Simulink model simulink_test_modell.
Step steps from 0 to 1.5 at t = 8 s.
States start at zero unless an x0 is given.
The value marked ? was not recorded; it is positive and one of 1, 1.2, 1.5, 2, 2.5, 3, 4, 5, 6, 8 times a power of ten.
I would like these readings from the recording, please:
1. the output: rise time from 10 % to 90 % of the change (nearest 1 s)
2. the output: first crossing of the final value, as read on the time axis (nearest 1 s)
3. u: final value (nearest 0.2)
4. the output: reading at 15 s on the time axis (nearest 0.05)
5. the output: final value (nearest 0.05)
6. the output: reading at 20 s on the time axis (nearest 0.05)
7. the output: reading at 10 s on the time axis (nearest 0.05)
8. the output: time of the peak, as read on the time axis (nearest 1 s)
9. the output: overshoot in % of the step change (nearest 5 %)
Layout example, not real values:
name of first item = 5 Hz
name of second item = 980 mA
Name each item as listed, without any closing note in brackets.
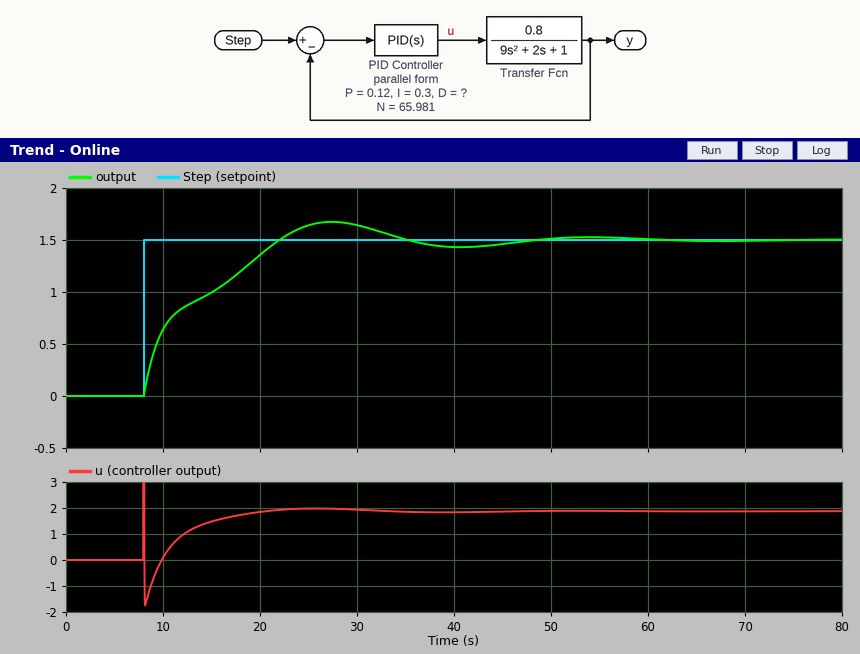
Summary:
the output: rise time from 10 % to 90 % of the change = 12 s
the output: first crossing of the final value, as read on the time axis = 22 s
u: final value = 1.8
the output: reading at 15 s on the time axis = 1.00
the output: final value = 1.50
the output: reading at 20 s on the time axis = 1.35
the output: reading at 10 s on the time axis = 0.65
the output: time of the peak, as read on the time axis = 27 s
the output: overshoot in % of the step change = 10 %
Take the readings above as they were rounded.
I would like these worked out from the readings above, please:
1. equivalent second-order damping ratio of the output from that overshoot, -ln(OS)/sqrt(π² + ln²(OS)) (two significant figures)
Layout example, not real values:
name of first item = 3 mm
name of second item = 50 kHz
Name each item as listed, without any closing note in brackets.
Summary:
equivalent second-order damping ratio of the output from that overshoot, -ln(OS)/sqrt(π² + ln²(OS)) = 0.59
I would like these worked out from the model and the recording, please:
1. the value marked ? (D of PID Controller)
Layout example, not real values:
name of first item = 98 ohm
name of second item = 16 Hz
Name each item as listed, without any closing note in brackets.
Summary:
the value marked ? = 4
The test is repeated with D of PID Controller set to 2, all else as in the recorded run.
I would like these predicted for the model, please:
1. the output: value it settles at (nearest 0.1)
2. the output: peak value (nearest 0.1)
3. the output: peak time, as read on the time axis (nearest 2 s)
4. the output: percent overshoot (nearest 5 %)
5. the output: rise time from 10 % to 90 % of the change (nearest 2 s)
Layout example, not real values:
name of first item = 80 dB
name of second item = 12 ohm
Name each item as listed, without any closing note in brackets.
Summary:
the output: value it settles at = 1.5
the output: peak value = 1.7
the output: peak time, as read on the time axis = 22 s
the output: percent overshoot = 15 %
the output: rise time from 10 % to 90 % of the change = 8 s
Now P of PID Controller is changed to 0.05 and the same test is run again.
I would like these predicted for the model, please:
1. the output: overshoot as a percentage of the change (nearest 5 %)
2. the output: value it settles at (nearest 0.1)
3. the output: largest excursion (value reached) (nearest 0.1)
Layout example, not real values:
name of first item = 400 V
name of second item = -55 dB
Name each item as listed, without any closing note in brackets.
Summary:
the output: overshoot as a percentage of the change = 15 %
the output: value it settles at = 1.5
the output: largest excursion (value reached) = 1.7
